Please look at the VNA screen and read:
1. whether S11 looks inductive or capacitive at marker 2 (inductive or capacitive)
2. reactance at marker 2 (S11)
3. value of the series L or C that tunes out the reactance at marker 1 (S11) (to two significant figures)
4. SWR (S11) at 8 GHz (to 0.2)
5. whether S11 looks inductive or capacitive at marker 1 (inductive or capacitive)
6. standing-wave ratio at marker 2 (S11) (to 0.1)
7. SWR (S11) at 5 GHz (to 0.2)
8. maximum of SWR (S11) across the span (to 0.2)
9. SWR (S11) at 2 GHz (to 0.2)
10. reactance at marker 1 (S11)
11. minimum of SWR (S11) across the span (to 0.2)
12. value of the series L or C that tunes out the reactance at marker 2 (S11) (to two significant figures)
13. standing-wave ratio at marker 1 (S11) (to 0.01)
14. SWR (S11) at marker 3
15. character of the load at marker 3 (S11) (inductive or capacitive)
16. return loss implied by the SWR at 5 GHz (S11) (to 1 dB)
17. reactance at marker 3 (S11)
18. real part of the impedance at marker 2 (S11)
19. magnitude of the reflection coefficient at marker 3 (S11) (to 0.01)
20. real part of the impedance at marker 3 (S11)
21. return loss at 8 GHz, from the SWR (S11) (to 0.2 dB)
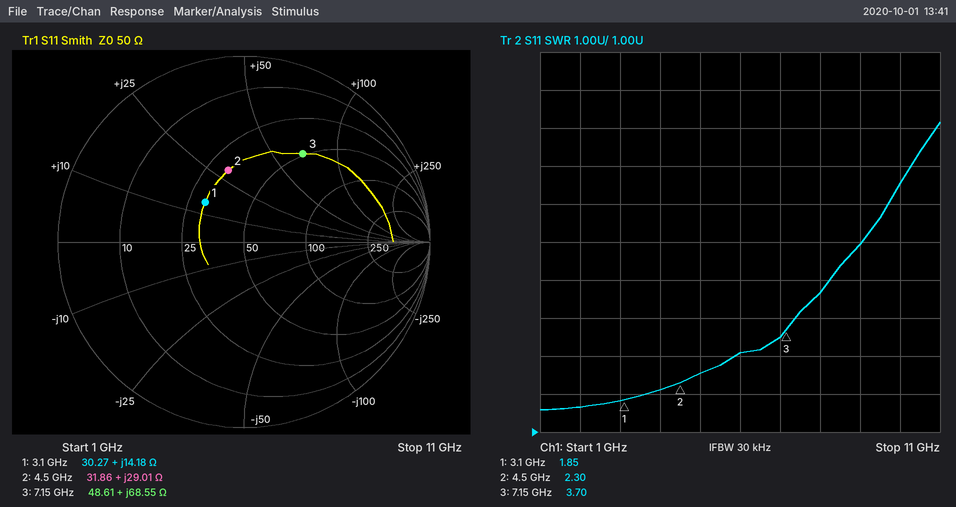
inductive
+29.01 Ω
3.6 pF
4.6
inductive
2.3
2.6
9.2
1.6
+14.18 Ω
1.6
1.2 pF
1.85
3.70
inductive
7 dB
+68.55 Ω
31.86 Ω
0.57
48.61 Ω
3.8 dB
